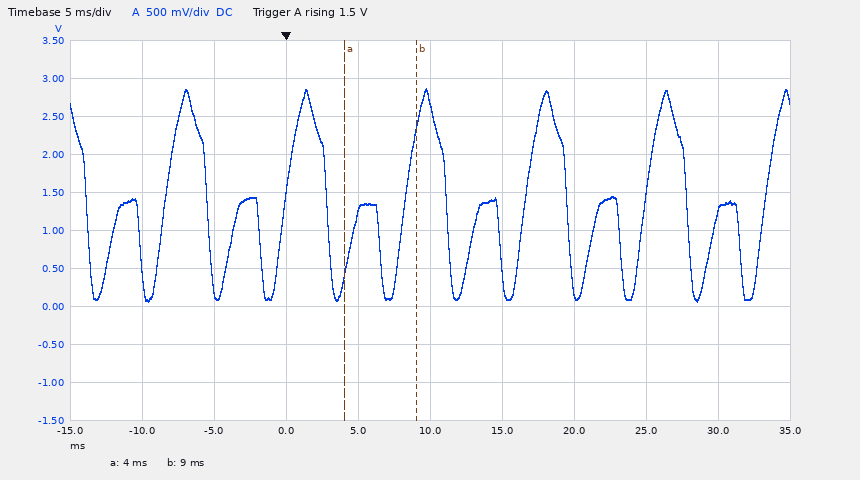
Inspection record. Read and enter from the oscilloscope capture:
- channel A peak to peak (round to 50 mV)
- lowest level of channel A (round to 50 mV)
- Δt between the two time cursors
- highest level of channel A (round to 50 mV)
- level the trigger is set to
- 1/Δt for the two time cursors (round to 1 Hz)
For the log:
2.80 V
50 mV
5.0 ms
2.85 V
1.5 V
200 Hz
